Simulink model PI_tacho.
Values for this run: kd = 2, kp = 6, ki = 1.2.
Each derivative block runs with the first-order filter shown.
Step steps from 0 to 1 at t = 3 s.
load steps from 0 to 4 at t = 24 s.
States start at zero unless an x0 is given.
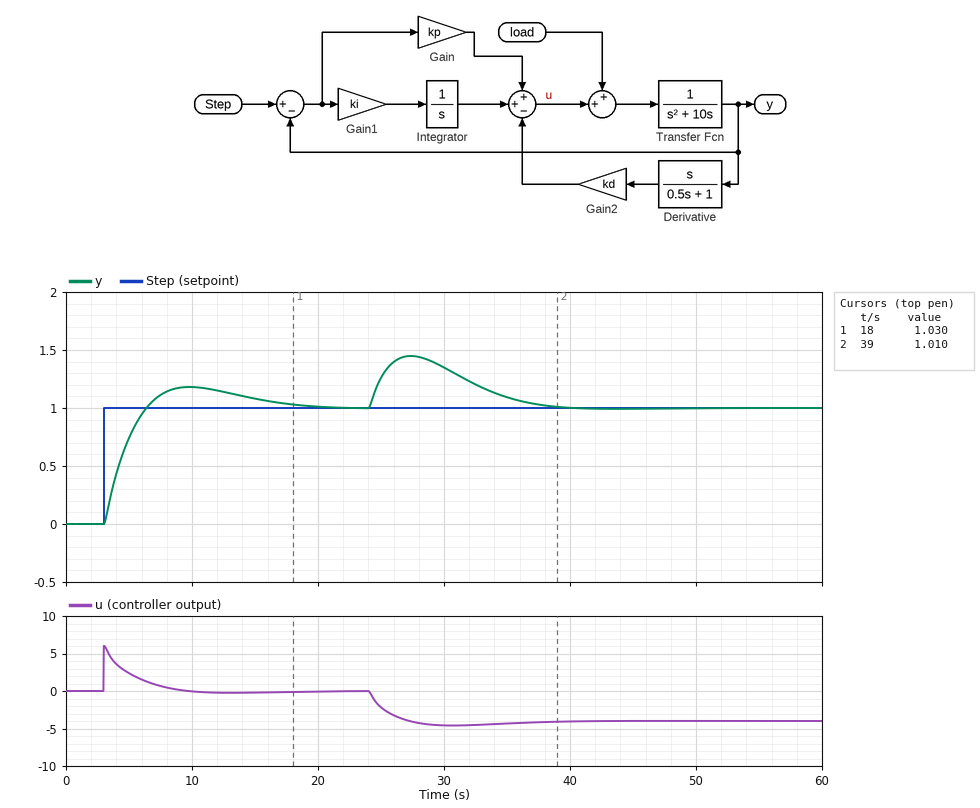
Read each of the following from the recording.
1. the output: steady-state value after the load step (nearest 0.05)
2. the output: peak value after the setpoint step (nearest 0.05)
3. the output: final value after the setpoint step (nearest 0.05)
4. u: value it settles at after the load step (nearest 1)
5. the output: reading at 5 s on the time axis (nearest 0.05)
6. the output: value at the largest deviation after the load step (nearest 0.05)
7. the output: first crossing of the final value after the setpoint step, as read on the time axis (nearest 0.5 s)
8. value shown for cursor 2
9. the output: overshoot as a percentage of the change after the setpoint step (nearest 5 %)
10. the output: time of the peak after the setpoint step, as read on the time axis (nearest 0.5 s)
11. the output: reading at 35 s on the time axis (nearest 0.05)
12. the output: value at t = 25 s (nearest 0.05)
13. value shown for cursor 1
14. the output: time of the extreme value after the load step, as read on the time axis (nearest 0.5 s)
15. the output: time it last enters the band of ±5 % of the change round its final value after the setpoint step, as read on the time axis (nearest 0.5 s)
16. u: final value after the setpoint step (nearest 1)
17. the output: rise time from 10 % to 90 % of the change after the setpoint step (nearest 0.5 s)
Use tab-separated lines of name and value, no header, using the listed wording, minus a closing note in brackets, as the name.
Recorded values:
the output: steady-state value after the load step	1.00
the output: peak value after the setpoint step	1.20
the output: final value after the setpoint step	1.00
u: value it settles at after the load step	-4
the output: reading at 5 s on the time axis	0.75
the output: value at the largest deviation after the load step	1.45
the output: first crossing of the final value after the setpoint step, as read on the time axis	6.5 s
value shown for cursor 2	1.010
the output: overshoot as a percentage of the change after the setpoint step	20 %
the output: time of the peak after the setpoint step, as read on the time axis	10.0 s
the output: reading at 35 s on the time axis	1.10
the output: value at t = 25 s	1.25
value shown for cursor 1	1.030
the output: time of the extreme value after the load step, as read on the time axis	27.5 s
the output: time it last enters the band of ±5 % of the change round its final value after the setpoint step, as read on the time axis	16.5 s
u: final value after the setpoint step	0
the output: rise time from 10 % to 90 % of the change after the setpoint step	2.5 s
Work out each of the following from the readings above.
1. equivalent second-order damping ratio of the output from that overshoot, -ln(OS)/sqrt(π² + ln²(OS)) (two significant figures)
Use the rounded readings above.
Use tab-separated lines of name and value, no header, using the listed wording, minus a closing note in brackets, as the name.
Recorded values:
equivalent second-order damping ratio of the output from that overshoot, -ln(OS)/sqrt(π² + ln²(OS))	0.46
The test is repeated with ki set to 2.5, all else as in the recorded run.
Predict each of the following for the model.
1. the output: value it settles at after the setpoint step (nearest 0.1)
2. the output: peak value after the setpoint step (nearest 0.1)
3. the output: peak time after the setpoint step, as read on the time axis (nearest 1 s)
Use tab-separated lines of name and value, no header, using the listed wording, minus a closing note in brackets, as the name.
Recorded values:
the output: value it settles at after the setpoint step	1.0
the output: peak value after the setpoint step	1.3
the output: peak time after the setpoint step, as read on the time axis	8 s
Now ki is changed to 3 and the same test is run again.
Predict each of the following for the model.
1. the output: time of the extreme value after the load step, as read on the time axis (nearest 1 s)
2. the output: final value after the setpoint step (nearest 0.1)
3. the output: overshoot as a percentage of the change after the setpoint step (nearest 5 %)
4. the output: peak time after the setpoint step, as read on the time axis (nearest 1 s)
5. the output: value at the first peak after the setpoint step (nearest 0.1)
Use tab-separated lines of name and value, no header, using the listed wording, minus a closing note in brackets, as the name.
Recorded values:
the output: time of the extreme value after the load step, as read on the time axis	26 s
the output: final value after the setpoint step	1.0
the output: overshoot as a percentage of the change after the setpoint step	30 %
the output: peak time after the setpoint step, as read on the time axis	8 s
the output: value at the first peak after the setpoint step	1.3
